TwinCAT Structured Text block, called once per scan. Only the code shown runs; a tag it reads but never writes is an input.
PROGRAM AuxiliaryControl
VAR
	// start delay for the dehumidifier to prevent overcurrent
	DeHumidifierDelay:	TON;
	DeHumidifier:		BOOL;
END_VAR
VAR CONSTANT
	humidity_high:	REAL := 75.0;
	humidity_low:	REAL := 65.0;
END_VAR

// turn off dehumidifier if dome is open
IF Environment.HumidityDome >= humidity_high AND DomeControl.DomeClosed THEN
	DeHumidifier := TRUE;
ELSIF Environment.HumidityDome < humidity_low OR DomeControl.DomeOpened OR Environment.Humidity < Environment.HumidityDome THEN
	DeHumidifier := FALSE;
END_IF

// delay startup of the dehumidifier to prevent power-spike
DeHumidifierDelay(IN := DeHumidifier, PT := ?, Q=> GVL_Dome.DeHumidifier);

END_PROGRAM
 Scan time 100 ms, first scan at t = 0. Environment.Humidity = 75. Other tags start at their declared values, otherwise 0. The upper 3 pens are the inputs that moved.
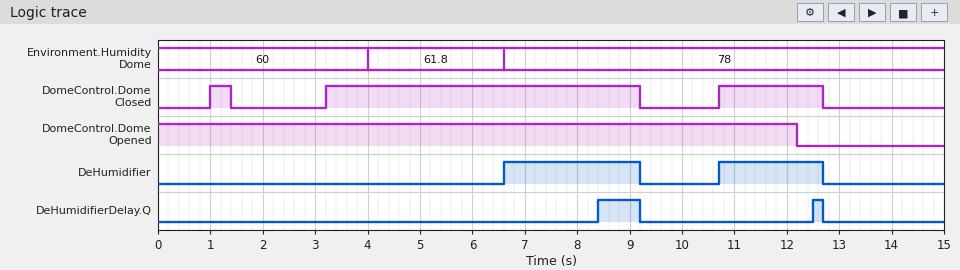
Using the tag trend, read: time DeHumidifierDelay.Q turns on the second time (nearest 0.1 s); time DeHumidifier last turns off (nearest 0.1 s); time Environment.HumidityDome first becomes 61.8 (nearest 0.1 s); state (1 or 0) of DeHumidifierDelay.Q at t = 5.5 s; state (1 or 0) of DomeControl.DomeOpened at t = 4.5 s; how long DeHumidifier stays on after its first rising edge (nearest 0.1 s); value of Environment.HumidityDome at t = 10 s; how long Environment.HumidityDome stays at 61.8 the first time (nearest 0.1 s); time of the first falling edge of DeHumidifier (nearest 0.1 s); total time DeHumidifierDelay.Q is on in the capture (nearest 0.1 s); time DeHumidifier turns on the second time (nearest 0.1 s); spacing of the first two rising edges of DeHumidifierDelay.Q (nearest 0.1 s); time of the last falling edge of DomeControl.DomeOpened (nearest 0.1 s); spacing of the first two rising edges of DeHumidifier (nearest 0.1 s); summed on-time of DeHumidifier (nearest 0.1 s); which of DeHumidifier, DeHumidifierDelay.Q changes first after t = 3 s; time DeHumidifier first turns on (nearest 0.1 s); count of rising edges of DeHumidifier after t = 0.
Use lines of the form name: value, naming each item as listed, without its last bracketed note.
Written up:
time DeHumidifierDelay.Q turns on the second time: 12.5 s
time DeHumidifier last turns off: 12.7 s
time Environment.HumidityDome first becomes 61.8: 4.0 s
state (1 or 0) of DeHumidifierDelay.Q at t = 5.5 s: 0
state (1 or 0) of DomeControl.DomeOpened at t = 4.5 s: 1
how long DeHumidifier stays on after its first rising edge: 2.6 s
value of Environment.HumidityDome at t = 10 s: 78
how long Environment.HumidityDome stays at 61.8 the first time: 2.6 s
time of the first falling edge of DeHumidifier: 9.2 s
total time DeHumidifierDelay.Q is on in the capture: 1.0 s
time DeHumidifier turns on the second time: 10.7 s
spacing of the first two rising edges of DeHumidifierDelay.Q: 4.1 s
time of the last falling edge of DomeControl.DomeOpened: 12.2 s
spacing of the first two rising edges of DeHumidifier: 4.1 s
summed on-time of DeHumidifier: 4.6 s
which of DeHumidifier, DeHumidifierDelay.Q changes first after t = 3 s: DeHumidifier
time DeHumidifier first turns on: 6.6 s
count of rising edges of DeHumidifier after t = 0: 2
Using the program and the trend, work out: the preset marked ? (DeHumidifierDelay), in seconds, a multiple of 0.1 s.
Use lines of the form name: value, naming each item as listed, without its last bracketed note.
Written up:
the preset marked ? (DeHumidifierDelay), in seconds, a multiple of 0.1 s: 1.8 s
